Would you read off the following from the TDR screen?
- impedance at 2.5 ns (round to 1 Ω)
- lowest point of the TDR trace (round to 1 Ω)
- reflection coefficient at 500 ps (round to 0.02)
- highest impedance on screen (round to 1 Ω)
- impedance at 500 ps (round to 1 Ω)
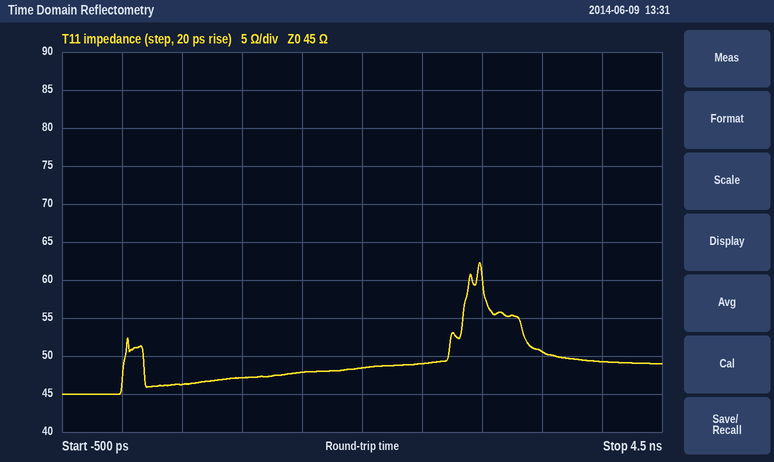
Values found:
49 Ω
45 Ω
+0.02
62 Ω
46 Ω
